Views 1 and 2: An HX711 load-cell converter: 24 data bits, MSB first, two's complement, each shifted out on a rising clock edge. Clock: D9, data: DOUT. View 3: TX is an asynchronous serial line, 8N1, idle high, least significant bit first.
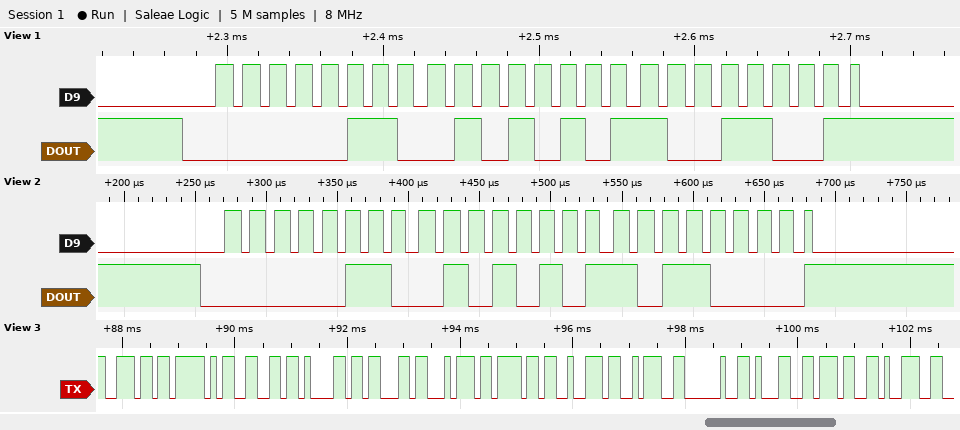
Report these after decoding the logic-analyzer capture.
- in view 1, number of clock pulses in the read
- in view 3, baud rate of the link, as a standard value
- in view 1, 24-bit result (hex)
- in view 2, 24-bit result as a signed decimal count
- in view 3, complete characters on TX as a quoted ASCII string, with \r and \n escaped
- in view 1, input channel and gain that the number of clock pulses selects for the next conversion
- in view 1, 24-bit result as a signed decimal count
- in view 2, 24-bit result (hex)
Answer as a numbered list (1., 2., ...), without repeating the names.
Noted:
1. 25
2. 9600 baud
3. 0x065599
4. 415152
5. "n_factor: 179"
6. channel A, gain 128
7. 415129
8. 0x0655B0
